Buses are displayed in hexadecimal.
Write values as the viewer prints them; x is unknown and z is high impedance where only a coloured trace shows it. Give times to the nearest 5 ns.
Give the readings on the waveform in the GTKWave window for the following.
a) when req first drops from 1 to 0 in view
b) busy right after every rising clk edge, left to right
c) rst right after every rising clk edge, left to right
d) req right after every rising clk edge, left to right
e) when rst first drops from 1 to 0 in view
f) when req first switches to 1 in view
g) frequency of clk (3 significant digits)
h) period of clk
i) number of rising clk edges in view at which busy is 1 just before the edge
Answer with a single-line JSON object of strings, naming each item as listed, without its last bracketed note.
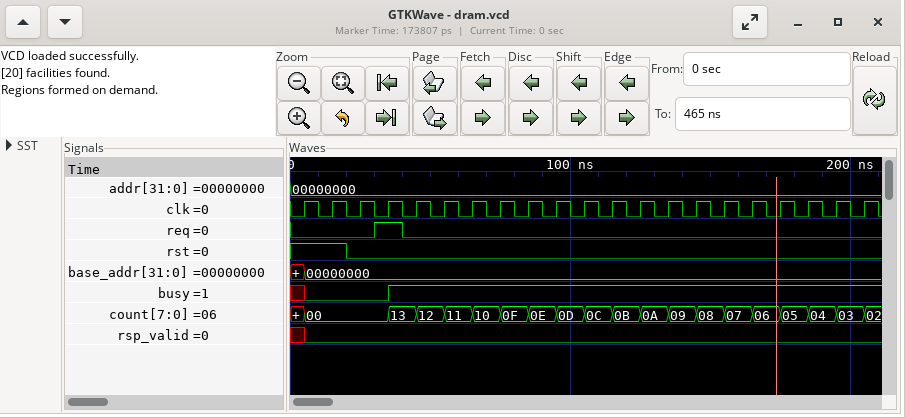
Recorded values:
{"when req first drops from 1 to 0 in view": "40 ns", "busy right after every rising clk edge, left to right": "0 0 0 1 1 1 1 1 1 1 1 1 1 1 1 1 1 1 1 1 1", "rst right after every rising clk edge, left to right": "1 1 0 0 0 0 0 0 0 0 0 0 0 0 0 0 0 0 0 0 0", "req right after every rising clk edge, left to right": "0 0 0 1 0 0 0 0 0 0 0 0 0 0 0 0 0 0 0 0 0", "when rst first drops from 1 to 0 in view": "20 ns", "when req first switches to 1 in view": "30 ns", "frequency of clk": "100 MHz", "period of clk": "10 ns", "number of rising clk edges in view at which busy is 1 just before the edge": "17"}
